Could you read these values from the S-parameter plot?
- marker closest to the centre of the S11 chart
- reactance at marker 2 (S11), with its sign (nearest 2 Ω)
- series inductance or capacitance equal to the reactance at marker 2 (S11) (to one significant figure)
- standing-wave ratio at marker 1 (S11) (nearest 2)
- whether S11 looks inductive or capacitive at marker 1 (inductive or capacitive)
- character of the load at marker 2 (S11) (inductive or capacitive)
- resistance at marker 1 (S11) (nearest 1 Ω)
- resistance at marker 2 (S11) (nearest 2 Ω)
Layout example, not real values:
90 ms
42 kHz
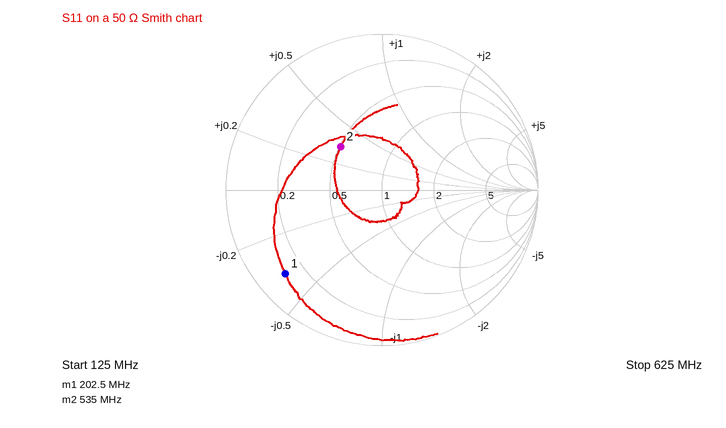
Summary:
marker 2
+16 Ω
5 nH
10
capacitive
inductive
6 Ω
26 Ω
